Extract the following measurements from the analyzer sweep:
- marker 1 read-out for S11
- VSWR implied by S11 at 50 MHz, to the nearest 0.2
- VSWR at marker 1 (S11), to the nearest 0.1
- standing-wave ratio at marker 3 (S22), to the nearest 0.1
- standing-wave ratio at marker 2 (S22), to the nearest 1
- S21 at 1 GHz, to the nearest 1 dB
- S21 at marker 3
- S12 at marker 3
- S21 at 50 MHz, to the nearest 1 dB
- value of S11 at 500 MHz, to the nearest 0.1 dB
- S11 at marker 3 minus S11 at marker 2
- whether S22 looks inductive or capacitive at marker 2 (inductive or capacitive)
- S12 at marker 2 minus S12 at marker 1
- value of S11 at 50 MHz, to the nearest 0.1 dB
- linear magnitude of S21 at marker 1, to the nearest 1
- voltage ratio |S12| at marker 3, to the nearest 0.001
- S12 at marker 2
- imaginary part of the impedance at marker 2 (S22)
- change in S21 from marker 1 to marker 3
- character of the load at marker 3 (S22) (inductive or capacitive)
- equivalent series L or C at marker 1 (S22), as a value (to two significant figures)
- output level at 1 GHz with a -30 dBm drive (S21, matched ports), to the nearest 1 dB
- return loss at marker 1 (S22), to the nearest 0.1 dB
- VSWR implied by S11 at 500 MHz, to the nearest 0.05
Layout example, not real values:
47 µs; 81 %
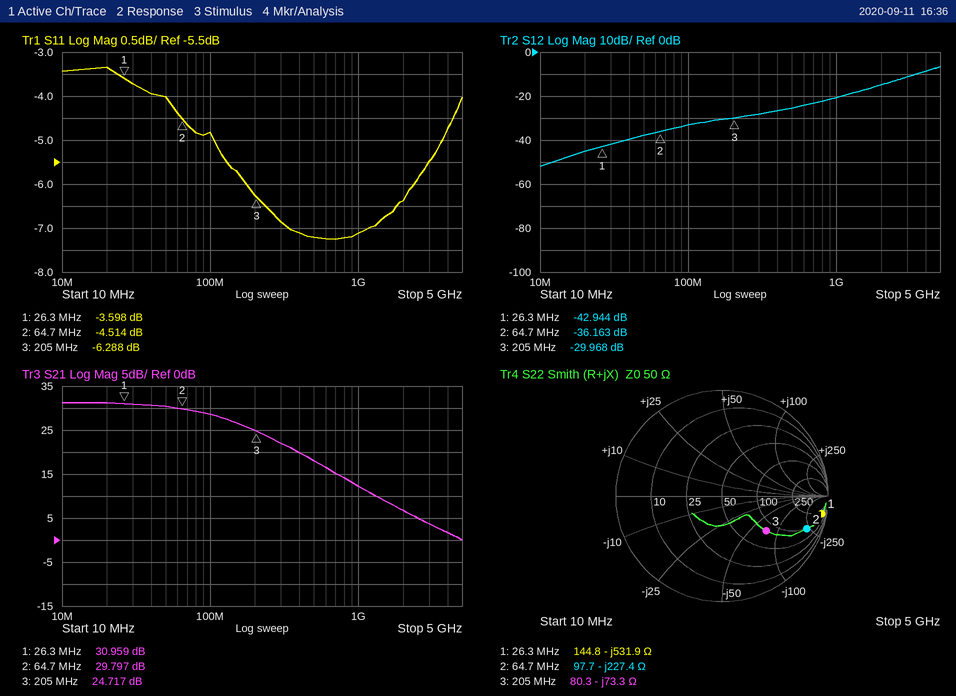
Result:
-3.598 dB; 4.4; 4.9; 3.3; 13; 12 dB; 24.717 dB; -29.968 dB; 30 dB; -7.2 dB; -1.774 dB; capacitive; 6.781 dB; -4.0 dB; 35; 0.032; -36.163 dB; -227.4 Ω; -6.242 dB; capacitive; 11 pF; -18 dBm; 0.4 dB; 2.55
